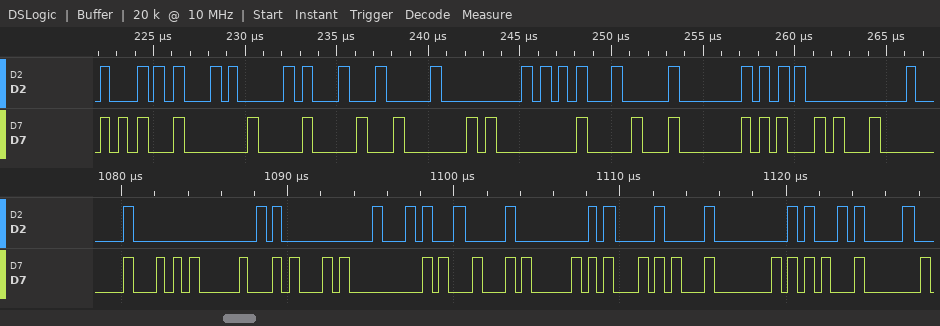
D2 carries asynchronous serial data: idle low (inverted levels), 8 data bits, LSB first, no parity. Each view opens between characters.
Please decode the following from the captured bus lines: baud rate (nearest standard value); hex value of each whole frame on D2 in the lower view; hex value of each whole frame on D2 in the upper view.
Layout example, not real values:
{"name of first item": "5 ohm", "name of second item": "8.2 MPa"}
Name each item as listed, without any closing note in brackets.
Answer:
{"baud rate": "2000000 baud", "hex value of each whole frame on D2 in the lower view": "FF, FD, D7, DF, 7D, FF, 5D", "hex value of each whole frame on D2 in the upper view": "57, 7D, 77, FF, D5, DF, D5"}
